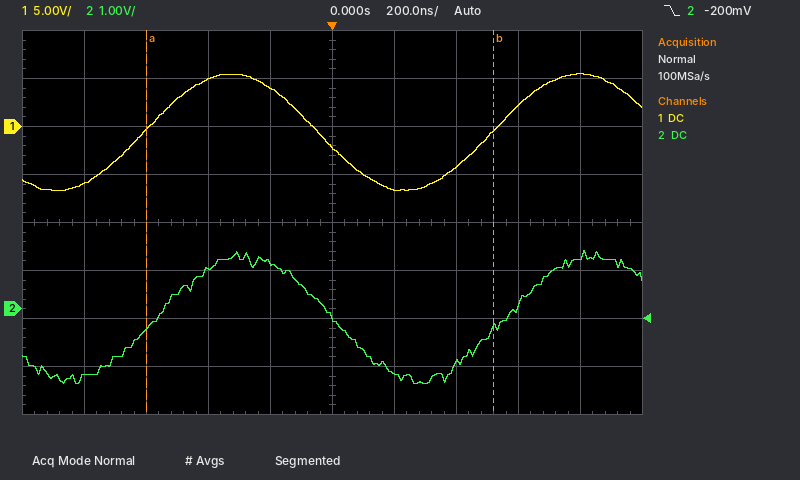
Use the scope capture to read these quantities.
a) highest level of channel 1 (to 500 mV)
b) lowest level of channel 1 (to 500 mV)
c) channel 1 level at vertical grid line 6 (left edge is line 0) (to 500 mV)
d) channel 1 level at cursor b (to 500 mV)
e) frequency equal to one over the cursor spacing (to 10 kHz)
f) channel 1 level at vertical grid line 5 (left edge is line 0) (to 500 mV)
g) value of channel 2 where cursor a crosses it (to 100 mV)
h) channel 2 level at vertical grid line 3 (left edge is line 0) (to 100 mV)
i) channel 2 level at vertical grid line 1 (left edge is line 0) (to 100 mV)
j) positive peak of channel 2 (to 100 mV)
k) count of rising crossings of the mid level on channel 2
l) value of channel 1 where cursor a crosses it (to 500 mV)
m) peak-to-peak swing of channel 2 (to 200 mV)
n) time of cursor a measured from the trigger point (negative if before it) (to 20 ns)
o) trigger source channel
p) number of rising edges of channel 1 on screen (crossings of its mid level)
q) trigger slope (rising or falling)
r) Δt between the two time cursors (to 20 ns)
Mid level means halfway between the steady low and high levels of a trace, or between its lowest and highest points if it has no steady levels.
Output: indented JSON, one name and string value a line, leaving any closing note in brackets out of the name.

{
  "highest level of channel 1": "5.5 V",
  "lowest level of channel 1": "-6.5 V",
  "channel 1 level at vertical grid line 6 (left edge is line 0)": "-6.5 V",
  "channel 1 level at cursor b": "-500 mV",
  "frequency equal to one over the cursor spacing": "890 kHz",
  "channel 1 level at vertical grid line 5 (left edge is line 0)": "-2.0 V",
  "value of channel 2 where cursor a crosses it": "-400 mV",
  "channel 2 level at vertical grid line 3 (left edge is line 0)": "800 mV",
  "channel 2 level at vertical grid line 1 (left edge is line 0)": "-1.4 V",
  "positive peak of channel 2": "1.2 V",
  "count of rising crossings of the mid level on channel 2": "2",
  "value of channel 1 where cursor a crosses it": "-500 mV",
  "peak-to-peak swing of channel 2": "2.8 V",
  "time of cursor a measured from the trigger point (negative if before it)": "-600 ns",
  "trigger source channel": "channel 2",
  "number of rising edges of channel 1 on screen": "2",
  "trigger slope": "falling",
  "Δt between the two time cursors": "1.12 µs"
}
